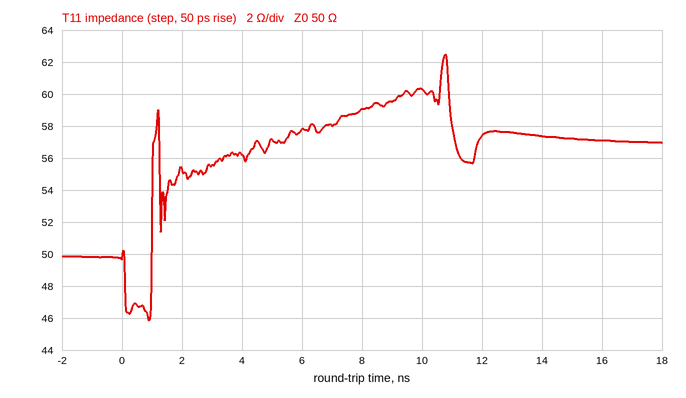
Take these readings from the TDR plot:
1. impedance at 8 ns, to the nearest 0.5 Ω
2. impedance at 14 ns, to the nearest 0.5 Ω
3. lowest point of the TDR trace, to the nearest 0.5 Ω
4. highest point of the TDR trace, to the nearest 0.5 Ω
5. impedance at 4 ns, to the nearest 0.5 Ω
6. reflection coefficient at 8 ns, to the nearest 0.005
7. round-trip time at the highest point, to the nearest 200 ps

59.0 Ω
57.5 Ω
46.0 Ω
62.5 Ω
56.0 Ω
+0.085
10.8 ns
